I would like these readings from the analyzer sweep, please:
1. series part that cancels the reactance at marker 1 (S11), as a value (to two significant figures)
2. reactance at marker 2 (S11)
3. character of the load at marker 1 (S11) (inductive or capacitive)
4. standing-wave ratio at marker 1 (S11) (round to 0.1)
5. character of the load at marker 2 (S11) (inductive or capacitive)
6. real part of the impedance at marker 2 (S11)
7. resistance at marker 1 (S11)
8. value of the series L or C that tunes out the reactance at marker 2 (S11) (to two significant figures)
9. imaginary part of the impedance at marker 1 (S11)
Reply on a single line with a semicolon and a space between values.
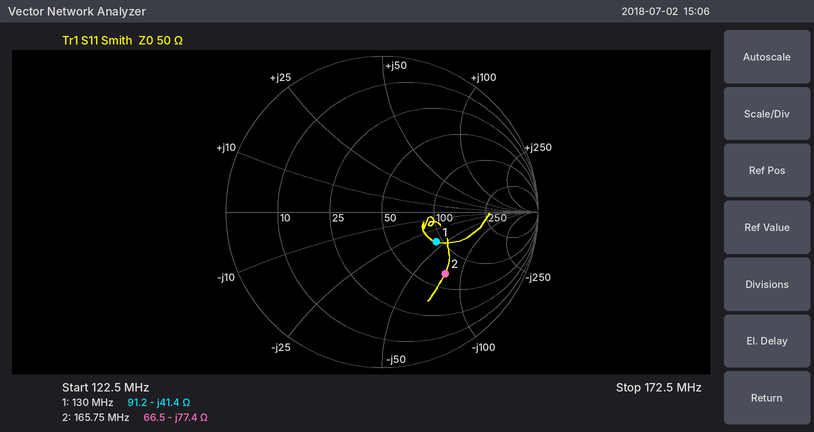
51 nH; -77.4 Ω; capacitive; 2.3; capacitive; 66.5 Ω; 91.2 Ω; 74 nH; -41.4 Ω
